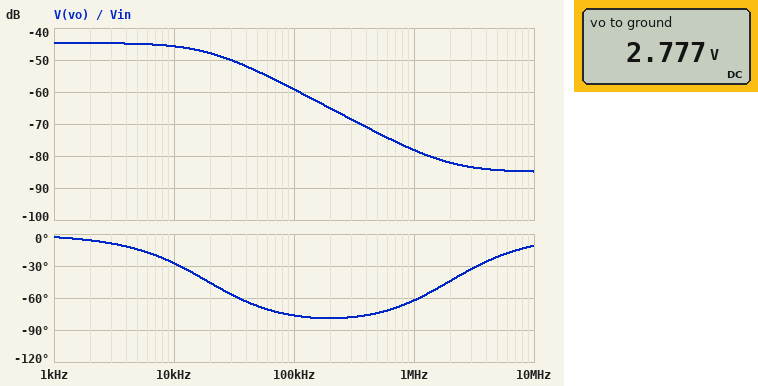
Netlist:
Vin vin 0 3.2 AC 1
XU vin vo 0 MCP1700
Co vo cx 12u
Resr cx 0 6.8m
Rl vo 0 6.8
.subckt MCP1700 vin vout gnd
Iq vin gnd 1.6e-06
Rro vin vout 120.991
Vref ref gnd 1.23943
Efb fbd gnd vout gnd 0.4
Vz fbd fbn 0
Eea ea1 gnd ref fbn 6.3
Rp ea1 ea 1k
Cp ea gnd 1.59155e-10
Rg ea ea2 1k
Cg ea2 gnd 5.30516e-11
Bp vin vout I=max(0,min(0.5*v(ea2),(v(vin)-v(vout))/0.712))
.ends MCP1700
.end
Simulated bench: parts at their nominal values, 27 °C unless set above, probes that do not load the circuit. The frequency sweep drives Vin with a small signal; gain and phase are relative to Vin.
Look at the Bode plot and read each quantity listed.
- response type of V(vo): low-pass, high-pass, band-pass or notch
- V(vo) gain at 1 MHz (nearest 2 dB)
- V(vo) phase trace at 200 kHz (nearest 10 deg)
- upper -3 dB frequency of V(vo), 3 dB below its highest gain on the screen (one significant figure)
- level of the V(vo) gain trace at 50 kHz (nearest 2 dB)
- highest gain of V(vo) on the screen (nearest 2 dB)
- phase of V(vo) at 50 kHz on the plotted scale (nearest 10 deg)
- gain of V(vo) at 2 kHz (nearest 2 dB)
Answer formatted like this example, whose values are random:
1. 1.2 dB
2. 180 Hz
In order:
1. low-pass
2. -78 dB
3. -80 deg
4. 20 kHz
5. -54 dB
6. -44 dB
7. -70 deg
8. -44 dB
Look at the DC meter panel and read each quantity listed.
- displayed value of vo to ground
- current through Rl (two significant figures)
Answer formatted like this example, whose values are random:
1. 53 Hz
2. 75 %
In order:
1. 2.777 V
2. 410 mA
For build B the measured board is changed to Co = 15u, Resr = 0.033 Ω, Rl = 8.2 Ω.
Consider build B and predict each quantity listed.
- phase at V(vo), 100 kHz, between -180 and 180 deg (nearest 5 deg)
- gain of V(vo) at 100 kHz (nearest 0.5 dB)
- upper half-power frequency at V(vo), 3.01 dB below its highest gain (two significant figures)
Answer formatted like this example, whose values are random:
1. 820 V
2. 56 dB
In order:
1. -65 deg
2. -61.0 dB
3. 14 kHz
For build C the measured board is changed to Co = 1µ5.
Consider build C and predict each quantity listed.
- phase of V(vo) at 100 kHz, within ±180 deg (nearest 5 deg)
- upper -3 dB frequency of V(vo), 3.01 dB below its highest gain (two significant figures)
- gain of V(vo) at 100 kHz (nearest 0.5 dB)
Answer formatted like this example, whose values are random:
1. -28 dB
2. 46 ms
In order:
1. -30 deg
2. 200 kHz
3. -45.5 dB
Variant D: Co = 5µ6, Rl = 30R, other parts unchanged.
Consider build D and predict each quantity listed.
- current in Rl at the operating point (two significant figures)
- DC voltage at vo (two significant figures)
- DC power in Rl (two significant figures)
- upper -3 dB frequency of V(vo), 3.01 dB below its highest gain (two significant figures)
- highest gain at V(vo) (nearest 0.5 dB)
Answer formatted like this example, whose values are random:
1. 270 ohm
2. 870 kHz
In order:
1. 100 mA
2. 3.0 V
3. 300 mW
4. 39 kHz
5. -44.0 dB
